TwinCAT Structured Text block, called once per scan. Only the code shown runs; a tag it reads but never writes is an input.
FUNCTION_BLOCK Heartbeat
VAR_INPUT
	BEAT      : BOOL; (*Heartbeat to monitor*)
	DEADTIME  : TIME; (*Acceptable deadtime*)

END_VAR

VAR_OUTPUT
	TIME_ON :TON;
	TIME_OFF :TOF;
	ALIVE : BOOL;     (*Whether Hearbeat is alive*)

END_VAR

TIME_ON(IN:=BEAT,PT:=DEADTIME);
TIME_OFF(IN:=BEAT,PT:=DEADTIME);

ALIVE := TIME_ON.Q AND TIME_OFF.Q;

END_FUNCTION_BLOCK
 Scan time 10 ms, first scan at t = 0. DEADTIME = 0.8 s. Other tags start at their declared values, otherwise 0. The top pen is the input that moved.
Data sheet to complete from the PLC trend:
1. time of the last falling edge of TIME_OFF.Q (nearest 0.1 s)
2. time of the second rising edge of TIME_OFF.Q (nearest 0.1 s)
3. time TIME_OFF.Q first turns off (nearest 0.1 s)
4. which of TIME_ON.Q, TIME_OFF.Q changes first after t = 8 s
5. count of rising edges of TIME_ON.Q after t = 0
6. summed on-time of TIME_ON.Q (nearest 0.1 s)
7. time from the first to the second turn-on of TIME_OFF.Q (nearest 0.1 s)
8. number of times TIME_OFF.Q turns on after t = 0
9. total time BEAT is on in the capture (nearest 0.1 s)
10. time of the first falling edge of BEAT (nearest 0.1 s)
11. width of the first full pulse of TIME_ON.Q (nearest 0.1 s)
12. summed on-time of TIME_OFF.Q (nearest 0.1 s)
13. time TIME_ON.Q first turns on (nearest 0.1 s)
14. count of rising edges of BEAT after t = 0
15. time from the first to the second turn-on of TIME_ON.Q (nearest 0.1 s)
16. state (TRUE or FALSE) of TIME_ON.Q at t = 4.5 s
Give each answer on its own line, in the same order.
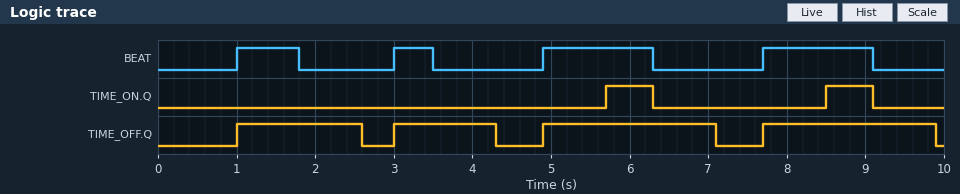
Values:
9.9 s
3.0 s
2.6 s
TIME_ON.Q
2
1.2 s
2.0 s
4
4.1 s
1.8 s
0.6 s
7.3 s
5.7 s
4
2.8 s
FALSE
